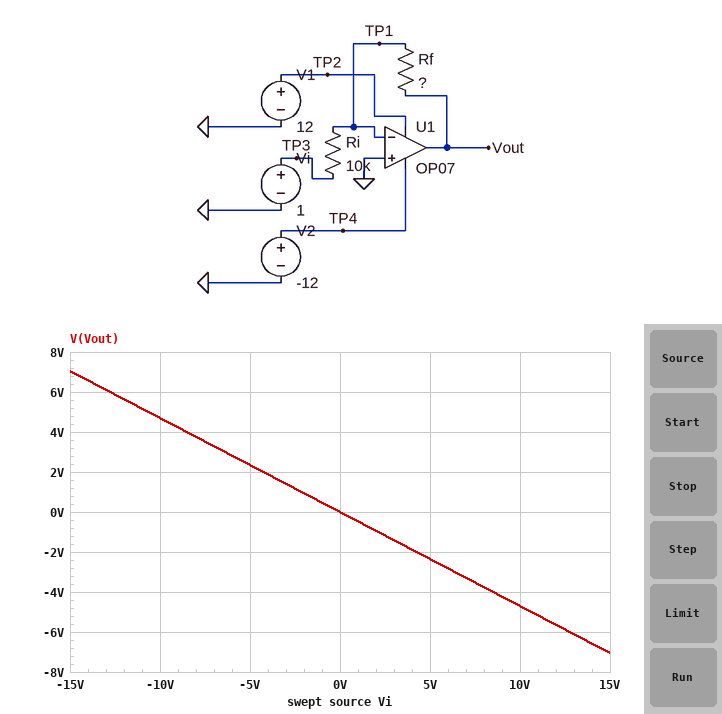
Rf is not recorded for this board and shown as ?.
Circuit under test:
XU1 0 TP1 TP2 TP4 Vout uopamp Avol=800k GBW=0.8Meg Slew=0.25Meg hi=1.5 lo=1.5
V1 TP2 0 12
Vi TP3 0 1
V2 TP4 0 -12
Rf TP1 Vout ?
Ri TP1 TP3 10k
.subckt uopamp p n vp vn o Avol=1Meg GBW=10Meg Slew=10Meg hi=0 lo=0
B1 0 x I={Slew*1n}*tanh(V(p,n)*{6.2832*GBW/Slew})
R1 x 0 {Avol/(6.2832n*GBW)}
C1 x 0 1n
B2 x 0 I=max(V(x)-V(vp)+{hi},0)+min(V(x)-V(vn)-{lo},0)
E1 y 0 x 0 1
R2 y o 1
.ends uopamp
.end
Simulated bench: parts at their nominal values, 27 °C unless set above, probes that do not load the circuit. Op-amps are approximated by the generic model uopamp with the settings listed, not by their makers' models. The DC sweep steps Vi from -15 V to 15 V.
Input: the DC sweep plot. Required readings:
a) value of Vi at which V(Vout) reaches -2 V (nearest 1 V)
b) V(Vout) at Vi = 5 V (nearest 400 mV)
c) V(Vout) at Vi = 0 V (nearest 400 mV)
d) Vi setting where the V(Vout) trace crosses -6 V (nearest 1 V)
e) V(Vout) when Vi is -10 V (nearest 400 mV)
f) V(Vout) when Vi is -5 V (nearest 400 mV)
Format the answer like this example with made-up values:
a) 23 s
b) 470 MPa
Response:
a) 4 V
b) -2.4 V
c) 0 V
d) 13 V
e) 4.8 V
f) 2.4 V
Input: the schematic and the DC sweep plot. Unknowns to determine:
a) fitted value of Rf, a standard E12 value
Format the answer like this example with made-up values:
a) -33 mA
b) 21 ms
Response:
a) 4.7 kΩ
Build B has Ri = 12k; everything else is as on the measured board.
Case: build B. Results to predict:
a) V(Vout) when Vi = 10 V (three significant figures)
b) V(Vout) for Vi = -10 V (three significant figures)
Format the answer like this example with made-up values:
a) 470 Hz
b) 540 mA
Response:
a) -3.92 V
b) 3.92 V
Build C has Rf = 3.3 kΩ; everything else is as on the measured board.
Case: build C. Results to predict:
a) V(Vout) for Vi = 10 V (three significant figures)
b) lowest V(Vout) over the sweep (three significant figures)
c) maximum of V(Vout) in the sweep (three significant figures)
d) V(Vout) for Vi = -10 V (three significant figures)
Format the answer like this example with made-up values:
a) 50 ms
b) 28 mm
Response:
a) -3.30 V
b) -4.95 V
c) 4.95 V
d) 3.30 V
